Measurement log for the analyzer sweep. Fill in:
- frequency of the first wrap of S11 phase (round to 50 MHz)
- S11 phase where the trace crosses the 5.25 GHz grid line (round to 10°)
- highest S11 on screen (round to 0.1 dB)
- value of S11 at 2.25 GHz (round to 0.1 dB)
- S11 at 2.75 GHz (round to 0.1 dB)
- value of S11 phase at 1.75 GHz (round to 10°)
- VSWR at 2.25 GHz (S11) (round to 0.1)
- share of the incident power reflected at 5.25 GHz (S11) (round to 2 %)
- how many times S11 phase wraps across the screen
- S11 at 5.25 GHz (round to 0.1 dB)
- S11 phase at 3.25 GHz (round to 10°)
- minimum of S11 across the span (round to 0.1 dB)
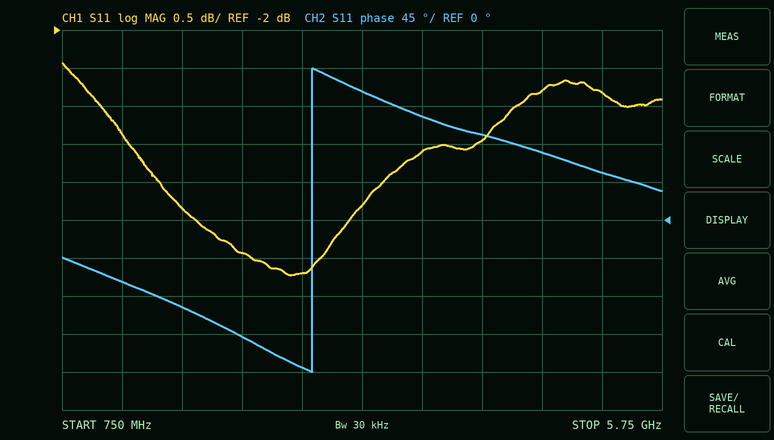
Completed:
2.85 GHz
60°
-2.4 dB
-4.9 dB
-5.2 dB
-100°
3.6
52 %
1
-2.8 dB
150°
-5.2 dB
